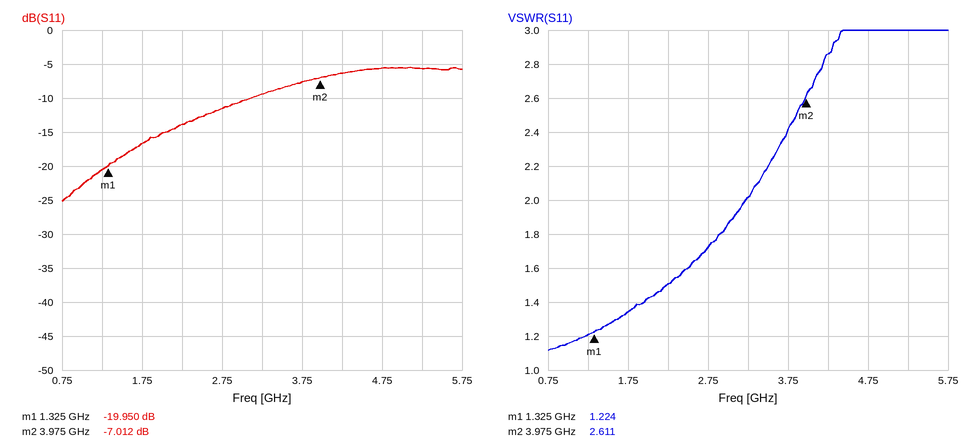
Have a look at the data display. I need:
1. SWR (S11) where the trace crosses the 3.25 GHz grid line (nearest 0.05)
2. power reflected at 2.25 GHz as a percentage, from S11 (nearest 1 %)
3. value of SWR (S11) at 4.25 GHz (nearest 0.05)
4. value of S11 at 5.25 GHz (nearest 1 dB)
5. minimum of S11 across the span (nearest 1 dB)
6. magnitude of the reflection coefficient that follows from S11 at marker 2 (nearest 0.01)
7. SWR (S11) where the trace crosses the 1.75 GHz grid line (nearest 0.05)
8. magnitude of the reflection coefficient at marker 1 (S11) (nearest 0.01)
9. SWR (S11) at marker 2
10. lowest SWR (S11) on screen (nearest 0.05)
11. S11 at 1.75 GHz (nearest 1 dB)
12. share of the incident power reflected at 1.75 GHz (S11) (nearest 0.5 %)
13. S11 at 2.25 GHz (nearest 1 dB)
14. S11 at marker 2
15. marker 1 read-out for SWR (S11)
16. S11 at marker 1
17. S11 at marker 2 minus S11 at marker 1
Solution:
2.00
4 %
2.85
-6 dB
-25 dB
0.45
1.35
0.10
2.611
1.10
-17 dB
2.0 %
-14 dB
-7.012 dB
1.224
-19.950 dB
12.938 dB
